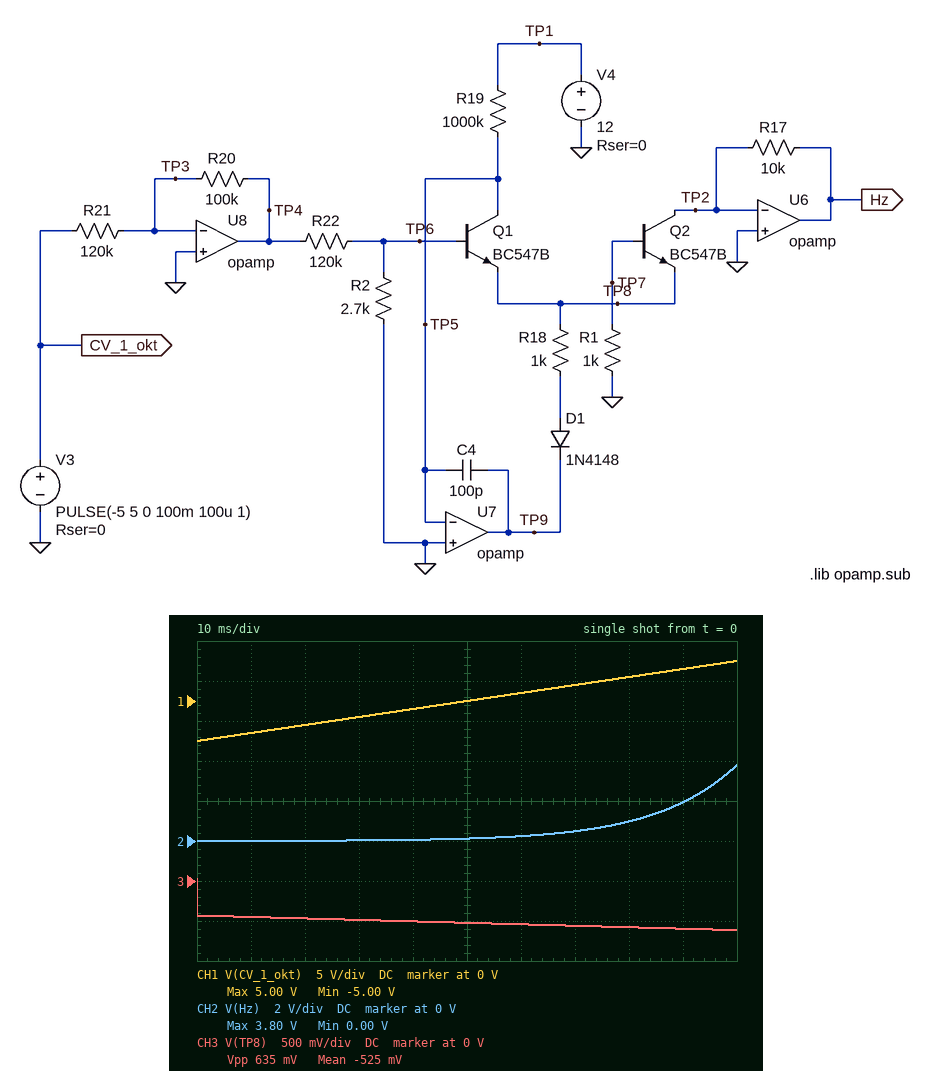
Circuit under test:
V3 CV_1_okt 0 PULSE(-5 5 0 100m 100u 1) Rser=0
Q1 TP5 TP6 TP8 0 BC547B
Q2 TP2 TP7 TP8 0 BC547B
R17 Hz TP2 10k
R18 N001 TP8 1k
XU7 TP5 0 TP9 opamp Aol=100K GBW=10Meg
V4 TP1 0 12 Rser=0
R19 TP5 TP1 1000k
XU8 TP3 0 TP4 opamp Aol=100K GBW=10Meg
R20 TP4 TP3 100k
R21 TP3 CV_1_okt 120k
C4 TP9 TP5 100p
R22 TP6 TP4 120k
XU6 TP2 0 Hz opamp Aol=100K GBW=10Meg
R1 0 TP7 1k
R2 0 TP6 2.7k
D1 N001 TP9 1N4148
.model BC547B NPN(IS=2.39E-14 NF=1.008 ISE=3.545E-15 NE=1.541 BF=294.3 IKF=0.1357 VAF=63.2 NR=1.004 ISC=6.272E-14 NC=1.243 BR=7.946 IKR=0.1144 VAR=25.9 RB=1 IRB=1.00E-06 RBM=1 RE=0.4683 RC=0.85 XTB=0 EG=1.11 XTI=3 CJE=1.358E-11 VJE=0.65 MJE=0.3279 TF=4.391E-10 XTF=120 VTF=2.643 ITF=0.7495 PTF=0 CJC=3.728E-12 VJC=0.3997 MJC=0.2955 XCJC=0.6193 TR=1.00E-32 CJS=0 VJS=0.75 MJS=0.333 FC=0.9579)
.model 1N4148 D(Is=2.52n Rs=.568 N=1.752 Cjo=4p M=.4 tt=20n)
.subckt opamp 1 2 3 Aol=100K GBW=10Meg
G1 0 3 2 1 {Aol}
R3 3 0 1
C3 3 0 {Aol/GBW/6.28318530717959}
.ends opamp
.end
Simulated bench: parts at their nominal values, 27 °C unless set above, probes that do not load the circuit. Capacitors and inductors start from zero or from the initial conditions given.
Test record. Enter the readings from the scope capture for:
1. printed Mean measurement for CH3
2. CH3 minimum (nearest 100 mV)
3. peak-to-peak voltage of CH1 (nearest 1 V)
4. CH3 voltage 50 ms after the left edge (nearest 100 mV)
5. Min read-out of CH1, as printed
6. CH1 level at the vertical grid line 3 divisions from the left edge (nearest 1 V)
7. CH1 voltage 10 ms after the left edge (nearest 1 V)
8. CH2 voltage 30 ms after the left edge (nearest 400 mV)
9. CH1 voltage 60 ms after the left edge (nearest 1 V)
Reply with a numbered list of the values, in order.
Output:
1. -525 mV
2. -600 mV
3. 10 V
4. -500 mV
5. -5.00 V
6. -2 V
7. -4 V
8. 0 V
9. 1 V
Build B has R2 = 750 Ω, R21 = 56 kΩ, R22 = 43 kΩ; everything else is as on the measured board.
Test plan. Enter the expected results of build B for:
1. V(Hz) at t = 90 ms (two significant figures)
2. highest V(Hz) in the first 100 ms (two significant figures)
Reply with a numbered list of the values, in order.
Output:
1. 11 V
2. 27 V
